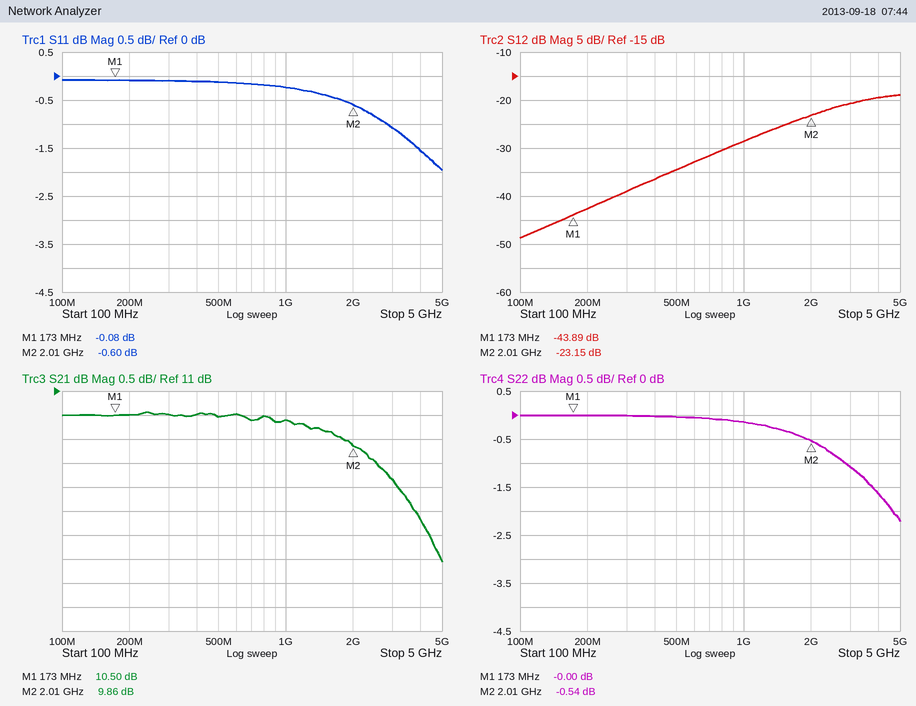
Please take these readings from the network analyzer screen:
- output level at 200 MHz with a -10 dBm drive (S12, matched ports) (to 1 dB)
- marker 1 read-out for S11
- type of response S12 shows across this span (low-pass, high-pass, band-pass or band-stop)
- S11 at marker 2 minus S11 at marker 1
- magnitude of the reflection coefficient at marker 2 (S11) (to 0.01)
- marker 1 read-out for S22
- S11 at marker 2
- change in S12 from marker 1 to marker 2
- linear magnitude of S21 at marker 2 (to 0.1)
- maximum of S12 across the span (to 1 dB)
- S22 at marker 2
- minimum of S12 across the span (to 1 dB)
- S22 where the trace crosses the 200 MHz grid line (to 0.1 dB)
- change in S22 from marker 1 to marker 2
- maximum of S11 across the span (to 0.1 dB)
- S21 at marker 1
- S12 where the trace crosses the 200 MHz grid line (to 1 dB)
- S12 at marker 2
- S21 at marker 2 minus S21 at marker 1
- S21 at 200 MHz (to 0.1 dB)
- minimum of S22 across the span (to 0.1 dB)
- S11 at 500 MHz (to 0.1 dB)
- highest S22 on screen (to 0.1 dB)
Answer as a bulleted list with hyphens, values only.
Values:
- -53 dBm
- -0.08 dB
- high-pass
- -0.52 dB
- 0.93
- -0.00 dB
- -0.60 dB
- 20.74 dB
- 3.1
- -19 dB
- -0.54 dB
- -49 dB
- 0.0 dB
- -0.54 dB
- -0.1 dB
- 10.50 dB
- -43 dB
- -23.15 dB
- -0.64 dB
- 10.5 dB
- -2.2 dB
- -0.1 dB
- 0.0 dB
